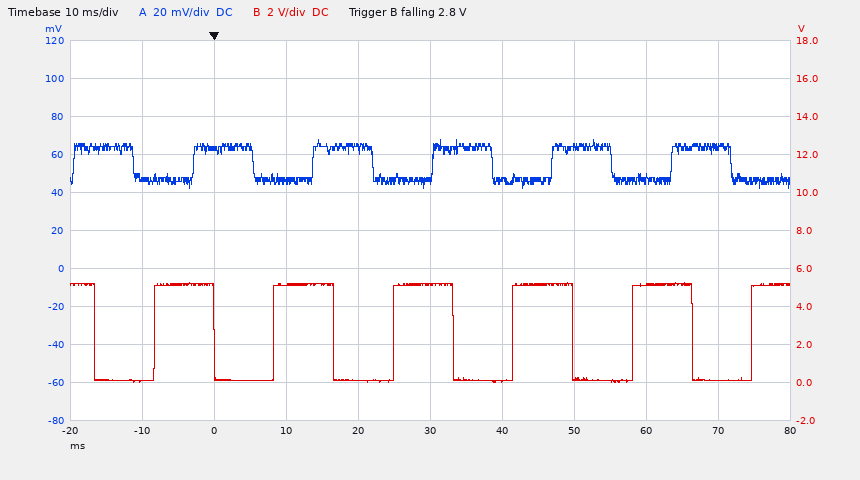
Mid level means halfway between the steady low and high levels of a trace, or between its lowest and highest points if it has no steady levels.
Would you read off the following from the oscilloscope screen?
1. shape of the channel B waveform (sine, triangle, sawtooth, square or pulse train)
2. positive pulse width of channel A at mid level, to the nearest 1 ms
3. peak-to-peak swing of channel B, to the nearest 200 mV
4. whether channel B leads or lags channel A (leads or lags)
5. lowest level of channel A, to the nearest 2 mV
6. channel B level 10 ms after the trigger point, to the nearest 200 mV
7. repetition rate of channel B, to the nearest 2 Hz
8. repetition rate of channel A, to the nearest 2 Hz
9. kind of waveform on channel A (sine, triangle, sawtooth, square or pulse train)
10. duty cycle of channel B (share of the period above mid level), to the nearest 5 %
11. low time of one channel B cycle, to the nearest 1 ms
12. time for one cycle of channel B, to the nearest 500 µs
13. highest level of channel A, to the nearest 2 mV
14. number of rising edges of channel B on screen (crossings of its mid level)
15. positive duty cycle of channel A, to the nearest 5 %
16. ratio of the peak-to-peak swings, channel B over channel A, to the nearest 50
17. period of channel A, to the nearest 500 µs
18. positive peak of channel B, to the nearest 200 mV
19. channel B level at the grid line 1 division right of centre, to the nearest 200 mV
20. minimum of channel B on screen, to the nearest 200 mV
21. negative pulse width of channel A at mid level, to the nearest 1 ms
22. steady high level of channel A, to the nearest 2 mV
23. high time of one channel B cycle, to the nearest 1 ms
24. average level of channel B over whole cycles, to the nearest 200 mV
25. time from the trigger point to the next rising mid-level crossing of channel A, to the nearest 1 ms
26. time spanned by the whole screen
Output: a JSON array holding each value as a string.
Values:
["square", "8 ms", "5.2 V", "leads", "42 mV", "5.2 V", "60 Hz", "60 Hz", "square", "50 %", "8 ms", "16.5 ms", "68 mV", "6", "50 %", "200", "16.5 ms", "5.2 V", "0.0 V", "0.0 V", "8 ms", "64 mV", "8 ms", "2.6 V", "14 ms", "100 ms"]
